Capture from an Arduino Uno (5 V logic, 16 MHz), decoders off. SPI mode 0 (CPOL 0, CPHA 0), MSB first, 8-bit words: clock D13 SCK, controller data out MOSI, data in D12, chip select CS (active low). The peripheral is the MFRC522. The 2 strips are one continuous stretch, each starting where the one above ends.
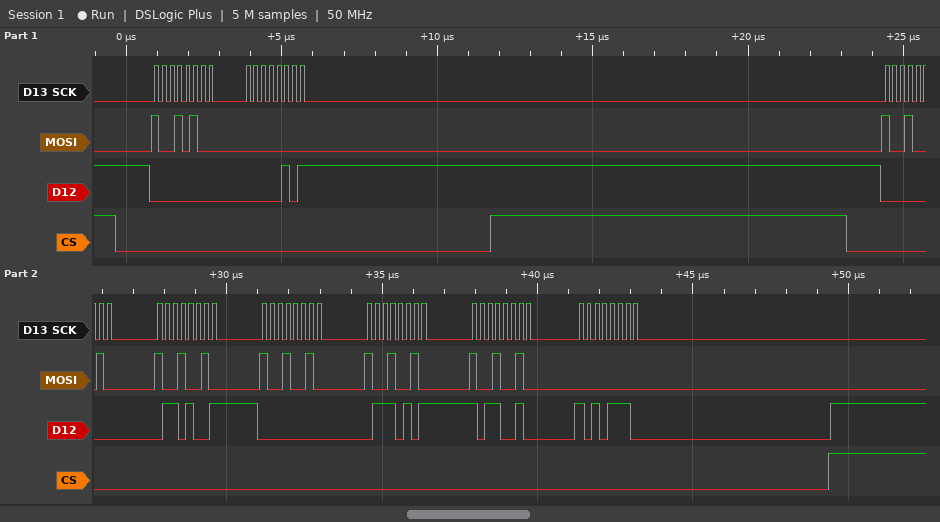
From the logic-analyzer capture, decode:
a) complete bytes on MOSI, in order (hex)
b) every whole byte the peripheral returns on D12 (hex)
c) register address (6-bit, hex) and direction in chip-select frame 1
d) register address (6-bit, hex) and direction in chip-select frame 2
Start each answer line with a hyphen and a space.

- 94 00 92 92 92 92 92 00
- 00 05 00 69 00 75 B2 AE
- 0x0A read
- 0x09 read
